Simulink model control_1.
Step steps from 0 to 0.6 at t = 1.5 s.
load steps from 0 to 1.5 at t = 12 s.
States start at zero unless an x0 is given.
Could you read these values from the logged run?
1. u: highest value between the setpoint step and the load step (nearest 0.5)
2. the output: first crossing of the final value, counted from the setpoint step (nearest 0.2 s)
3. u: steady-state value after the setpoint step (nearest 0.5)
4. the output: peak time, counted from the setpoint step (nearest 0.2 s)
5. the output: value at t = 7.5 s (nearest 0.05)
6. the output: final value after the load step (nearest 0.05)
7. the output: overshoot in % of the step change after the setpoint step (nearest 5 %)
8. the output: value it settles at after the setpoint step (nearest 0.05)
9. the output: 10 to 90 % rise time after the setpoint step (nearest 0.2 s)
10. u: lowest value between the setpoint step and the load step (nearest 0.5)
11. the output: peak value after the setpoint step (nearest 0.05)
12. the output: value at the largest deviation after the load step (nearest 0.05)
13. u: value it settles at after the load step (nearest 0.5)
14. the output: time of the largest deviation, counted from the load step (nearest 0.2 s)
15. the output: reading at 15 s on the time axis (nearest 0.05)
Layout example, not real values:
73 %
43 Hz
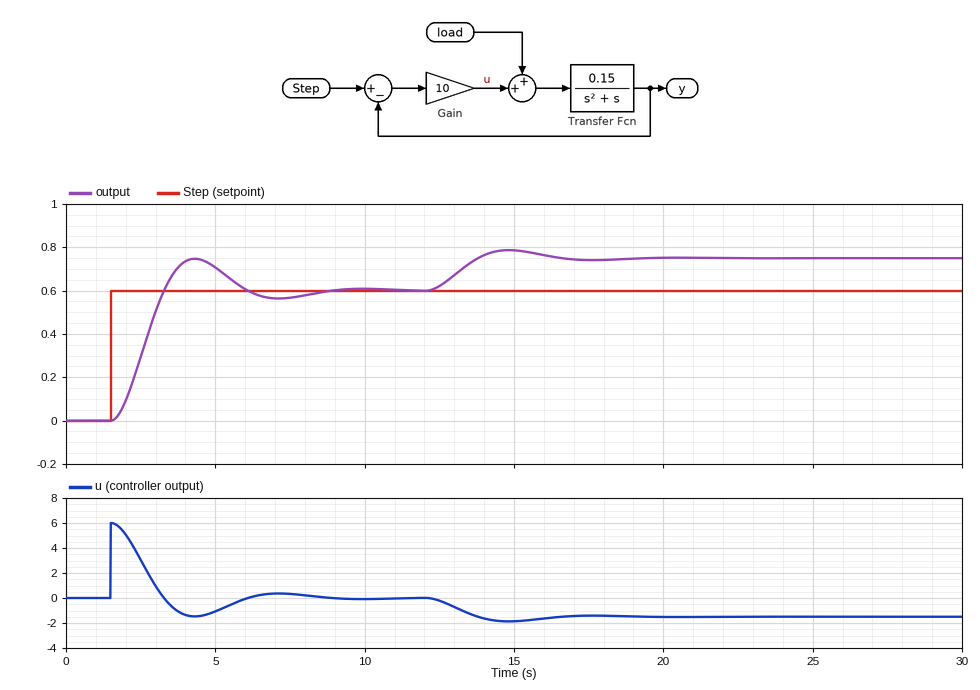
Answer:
6.0
1.8 s
0.0
2.8 s
0.55
0.75
25 %
0.60
1.2 s
-1.5
0.75
0.80
-1.5
2.8 s
0.80
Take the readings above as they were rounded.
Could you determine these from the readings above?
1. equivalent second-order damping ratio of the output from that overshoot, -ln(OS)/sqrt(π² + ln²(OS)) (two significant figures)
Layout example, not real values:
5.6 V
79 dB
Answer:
0.40
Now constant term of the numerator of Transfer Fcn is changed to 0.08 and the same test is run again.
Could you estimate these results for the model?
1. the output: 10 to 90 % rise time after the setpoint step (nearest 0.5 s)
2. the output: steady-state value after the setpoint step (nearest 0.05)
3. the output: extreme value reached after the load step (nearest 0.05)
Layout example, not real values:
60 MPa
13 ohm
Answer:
2.0 s
0.60
0.75
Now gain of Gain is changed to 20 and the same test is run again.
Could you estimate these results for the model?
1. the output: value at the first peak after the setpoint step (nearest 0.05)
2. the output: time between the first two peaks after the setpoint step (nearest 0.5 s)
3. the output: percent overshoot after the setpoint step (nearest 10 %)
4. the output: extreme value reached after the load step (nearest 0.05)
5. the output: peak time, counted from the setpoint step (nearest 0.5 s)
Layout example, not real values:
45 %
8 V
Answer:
0.85
4.0 s
40 %
0.70
2.0 s
